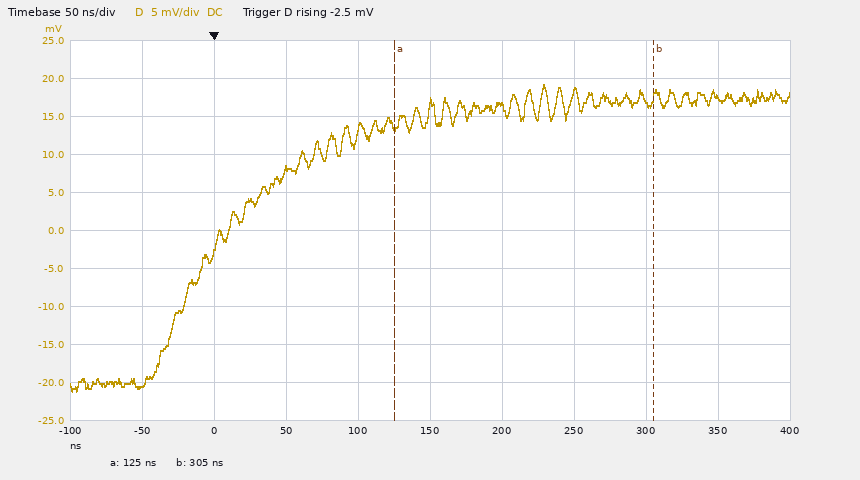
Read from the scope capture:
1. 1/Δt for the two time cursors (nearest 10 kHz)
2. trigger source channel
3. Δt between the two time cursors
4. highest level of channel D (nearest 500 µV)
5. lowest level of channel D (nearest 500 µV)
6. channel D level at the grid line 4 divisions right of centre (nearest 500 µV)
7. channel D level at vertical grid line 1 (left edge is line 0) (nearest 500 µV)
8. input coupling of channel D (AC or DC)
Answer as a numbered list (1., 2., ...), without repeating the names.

1. 5.56 MHz
2. channel D
3. 180 ns
4. 19.0 mV
5. -21.0 mV
6. 17.5 mV
7. -20.5 mV
8. DC
